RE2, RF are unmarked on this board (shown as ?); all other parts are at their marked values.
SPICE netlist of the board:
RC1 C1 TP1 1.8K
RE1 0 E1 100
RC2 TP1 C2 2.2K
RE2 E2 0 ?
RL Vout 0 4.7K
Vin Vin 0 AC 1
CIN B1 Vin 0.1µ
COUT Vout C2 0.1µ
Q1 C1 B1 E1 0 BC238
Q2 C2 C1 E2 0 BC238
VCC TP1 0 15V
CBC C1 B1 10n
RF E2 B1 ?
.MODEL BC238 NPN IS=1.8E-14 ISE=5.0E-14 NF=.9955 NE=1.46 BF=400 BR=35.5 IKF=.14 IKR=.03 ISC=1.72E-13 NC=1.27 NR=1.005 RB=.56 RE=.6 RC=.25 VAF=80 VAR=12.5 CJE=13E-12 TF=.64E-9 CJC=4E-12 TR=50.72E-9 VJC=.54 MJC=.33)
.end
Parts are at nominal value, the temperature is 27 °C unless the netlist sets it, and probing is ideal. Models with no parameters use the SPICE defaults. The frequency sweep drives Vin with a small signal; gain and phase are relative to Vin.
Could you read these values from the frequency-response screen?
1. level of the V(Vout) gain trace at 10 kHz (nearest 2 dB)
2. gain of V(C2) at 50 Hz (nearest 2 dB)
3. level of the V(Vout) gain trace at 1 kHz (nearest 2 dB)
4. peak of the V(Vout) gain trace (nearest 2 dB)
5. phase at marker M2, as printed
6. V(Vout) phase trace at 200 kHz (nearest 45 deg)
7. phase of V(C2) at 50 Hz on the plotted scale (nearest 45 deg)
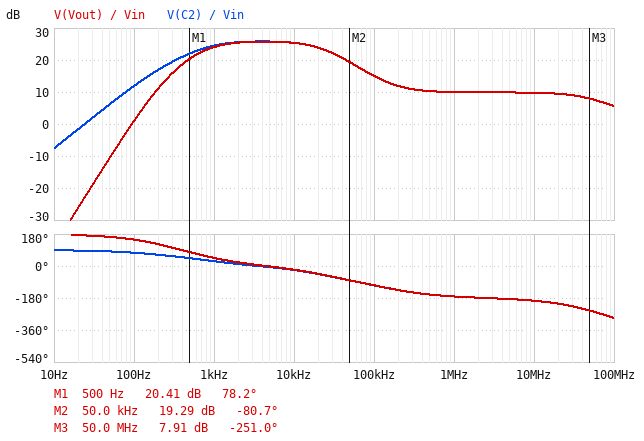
26 dB
6 dB
24 dB
26 dB
-80.7 deg
-135 deg
90 deg
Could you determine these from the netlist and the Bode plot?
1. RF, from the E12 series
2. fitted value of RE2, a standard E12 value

15 kΩ
470 Ω
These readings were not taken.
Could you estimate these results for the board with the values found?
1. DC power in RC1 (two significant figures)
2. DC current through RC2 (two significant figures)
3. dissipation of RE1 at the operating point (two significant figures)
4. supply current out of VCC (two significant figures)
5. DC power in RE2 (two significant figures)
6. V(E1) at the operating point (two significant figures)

88 mW
3.7 mA
4.9 mW
11 mA
6.5 mW
700 mV
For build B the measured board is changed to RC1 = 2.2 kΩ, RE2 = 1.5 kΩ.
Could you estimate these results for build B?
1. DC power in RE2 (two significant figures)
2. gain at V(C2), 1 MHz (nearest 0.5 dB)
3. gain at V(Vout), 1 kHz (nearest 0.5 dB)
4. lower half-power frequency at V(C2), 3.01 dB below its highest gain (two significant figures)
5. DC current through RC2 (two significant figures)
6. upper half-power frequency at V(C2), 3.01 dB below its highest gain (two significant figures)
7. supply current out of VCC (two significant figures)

1.6 mW
0 dB
15.0 dB
630 Hz
1.1 mA
24 kHz
6.9 mA
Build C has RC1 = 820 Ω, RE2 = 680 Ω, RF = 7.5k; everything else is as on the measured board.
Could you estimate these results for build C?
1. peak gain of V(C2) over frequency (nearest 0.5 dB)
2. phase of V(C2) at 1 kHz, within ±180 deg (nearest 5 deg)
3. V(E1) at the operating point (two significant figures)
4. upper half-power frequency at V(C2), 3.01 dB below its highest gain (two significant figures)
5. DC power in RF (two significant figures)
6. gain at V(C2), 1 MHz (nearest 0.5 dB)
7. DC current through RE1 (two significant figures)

20.0 dB
40 deg
1.4 V
40 kHz
18 µW
7.0 dB
14 mA
